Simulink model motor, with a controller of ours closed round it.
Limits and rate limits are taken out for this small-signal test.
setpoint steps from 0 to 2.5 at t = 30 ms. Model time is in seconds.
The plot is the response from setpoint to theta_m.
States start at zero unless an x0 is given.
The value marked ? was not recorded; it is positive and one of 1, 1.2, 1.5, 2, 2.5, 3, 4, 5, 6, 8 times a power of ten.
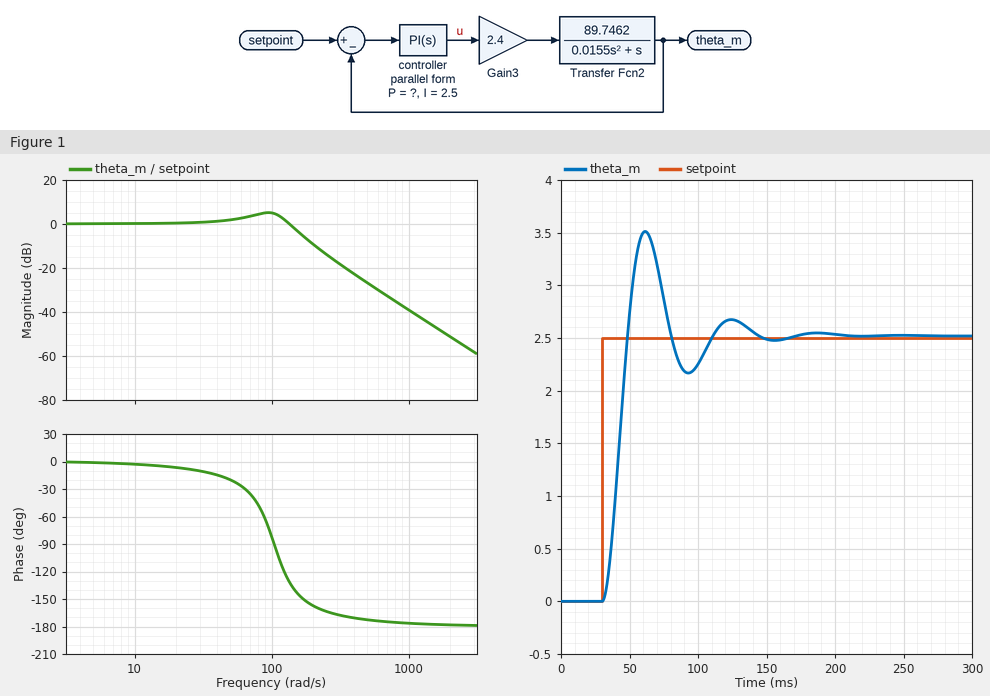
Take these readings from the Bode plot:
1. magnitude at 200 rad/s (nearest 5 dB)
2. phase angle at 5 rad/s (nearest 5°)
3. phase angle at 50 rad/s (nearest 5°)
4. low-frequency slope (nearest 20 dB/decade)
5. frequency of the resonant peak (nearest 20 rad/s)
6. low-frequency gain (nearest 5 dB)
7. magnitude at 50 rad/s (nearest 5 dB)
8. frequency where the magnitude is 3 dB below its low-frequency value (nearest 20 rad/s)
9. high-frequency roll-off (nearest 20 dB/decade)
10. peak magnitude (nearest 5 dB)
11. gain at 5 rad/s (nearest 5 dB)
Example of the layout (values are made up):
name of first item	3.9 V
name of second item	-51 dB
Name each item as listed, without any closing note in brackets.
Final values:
magnitude at 200 rad/s	-10 dB
phase angle at 5 rad/s	0°
phase angle at 50 rad/s	-20°
low-frequency slope	0 dB/decade
frequency of the resonant peak	100 rad/s
low-frequency gain	0 dB
magnitude at 50 rad/s	0 dB
frequency where the magnitude is 3 dB below its low-frequency value	160 rad/s
high-frequency roll-off	-40 dB/decade
peak magnitude	5 dB
gain at 5 rad/s	0 dB
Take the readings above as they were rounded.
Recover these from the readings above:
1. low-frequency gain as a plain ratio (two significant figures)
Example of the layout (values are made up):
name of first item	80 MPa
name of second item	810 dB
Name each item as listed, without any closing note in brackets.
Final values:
low-frequency gain as a plain ratio	1.0
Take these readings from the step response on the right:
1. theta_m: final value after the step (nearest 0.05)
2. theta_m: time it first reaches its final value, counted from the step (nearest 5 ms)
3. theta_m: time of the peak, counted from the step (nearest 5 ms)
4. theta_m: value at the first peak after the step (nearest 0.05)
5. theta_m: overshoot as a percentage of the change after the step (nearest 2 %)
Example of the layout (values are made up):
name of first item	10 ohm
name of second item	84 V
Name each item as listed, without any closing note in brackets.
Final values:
theta_m: final value after the step	2.50
theta_m: time it first reaches its final value, counted from the step	20 ms
theta_m: time of the peak, counted from the step	30 ms
theta_m: value at the first peak after the step	3.50
theta_m: overshoot as a percentage of the change after the step	40 %
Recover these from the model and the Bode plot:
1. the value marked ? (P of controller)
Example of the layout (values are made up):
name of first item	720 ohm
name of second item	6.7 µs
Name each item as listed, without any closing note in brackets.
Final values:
the value marked ?	0.8
